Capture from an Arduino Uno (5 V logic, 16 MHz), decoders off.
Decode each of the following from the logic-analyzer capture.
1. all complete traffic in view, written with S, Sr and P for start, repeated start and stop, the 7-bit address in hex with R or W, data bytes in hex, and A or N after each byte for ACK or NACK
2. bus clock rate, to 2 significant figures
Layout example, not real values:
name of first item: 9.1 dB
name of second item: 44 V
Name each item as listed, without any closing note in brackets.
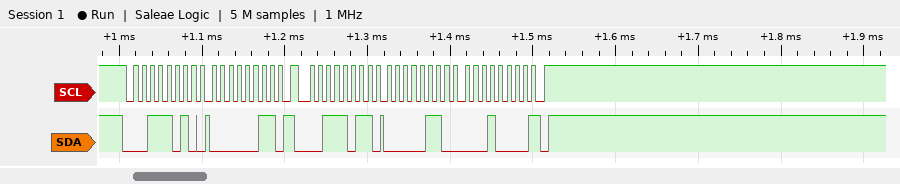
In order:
all complete traffic in view, written with S, Sr and P for start, repeated start and stop, the 7-bit address in hex with R or W, data bytes in hex, and A or N after each byte for ACK or NACK: S 1DW A 03 A Sr 1DR A 06 A 10 N P
bus clock rate, to 2 significant figures: 100 kHz
